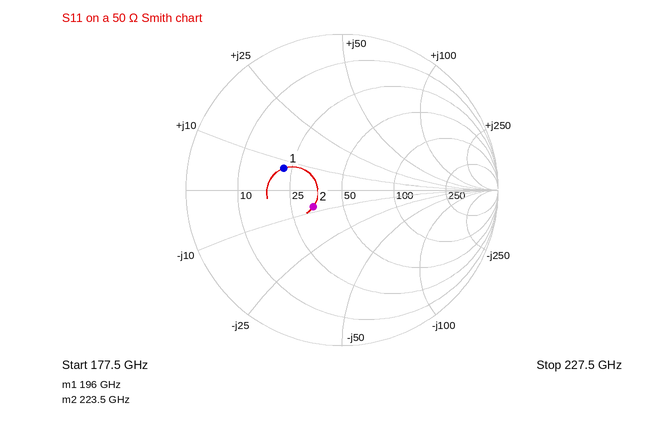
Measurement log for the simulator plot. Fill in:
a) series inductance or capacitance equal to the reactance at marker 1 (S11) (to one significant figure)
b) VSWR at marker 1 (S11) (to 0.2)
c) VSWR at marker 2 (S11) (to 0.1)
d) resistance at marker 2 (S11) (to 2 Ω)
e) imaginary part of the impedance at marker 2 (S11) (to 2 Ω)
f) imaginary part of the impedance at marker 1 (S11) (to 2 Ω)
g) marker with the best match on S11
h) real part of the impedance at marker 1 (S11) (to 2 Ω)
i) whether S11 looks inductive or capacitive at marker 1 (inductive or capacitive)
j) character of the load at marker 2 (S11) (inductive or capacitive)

6 pH
2.4
1.5
34 Ω
-8 Ω
+8 Ω
marker 2
22 Ω
inductive
capacitive
